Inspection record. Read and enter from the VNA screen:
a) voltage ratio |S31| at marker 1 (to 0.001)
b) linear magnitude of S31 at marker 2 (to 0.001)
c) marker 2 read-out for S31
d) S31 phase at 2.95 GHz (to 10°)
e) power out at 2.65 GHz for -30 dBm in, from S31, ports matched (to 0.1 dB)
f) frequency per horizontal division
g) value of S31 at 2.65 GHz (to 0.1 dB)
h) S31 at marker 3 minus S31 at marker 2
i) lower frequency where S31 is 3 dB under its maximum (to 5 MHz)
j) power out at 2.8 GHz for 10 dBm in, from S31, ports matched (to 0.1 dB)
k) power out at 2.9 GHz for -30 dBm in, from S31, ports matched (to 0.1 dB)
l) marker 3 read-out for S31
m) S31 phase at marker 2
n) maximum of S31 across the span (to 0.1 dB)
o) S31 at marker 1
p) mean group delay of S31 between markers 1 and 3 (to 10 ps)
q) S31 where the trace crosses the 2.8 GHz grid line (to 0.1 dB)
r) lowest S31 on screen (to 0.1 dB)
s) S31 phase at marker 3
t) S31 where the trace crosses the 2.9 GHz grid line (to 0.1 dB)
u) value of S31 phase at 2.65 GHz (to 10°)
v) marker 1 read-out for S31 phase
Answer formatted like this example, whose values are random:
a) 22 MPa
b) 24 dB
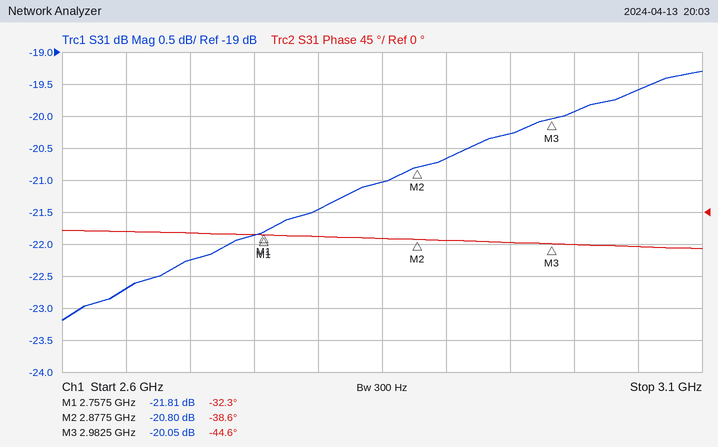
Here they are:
a) 0.081
b) 0.091
c) -20.80 dB
d) -40°
e) -52.7 dBm
f) 50 MHz
g) -22.7 dB
h) 0.75 dB
i) 2.695 GHz
j) -11.5 dBm
k) -50.7 dBm
l) -20.05 dB
m) -38.6°
n) -19.3 dB
o) -21.81 dB
p) 150 ps
q) -21.5 dB
r) -23.2 dB
s) -44.6°
t) -20.7 dB
u) -30°
v) -32.3°
